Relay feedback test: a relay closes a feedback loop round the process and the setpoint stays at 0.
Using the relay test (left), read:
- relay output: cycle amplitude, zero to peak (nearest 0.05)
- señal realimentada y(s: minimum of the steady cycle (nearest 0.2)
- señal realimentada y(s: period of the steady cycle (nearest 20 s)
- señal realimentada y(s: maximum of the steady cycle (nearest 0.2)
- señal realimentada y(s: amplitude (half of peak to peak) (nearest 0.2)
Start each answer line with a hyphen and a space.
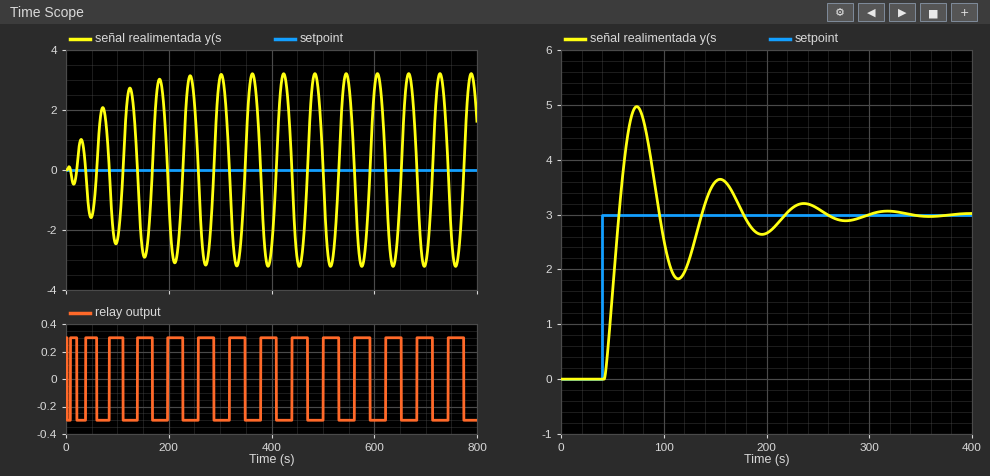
- 0.30
- -3.2
- 60 s
- 3.2
- 3.2
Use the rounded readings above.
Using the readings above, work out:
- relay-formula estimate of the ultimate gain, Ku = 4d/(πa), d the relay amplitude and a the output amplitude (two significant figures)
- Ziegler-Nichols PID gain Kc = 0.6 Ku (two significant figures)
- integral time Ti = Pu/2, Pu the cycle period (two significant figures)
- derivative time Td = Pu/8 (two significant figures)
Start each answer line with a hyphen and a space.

- 0.12
- 0.072
- 30 s
- 7.5 s
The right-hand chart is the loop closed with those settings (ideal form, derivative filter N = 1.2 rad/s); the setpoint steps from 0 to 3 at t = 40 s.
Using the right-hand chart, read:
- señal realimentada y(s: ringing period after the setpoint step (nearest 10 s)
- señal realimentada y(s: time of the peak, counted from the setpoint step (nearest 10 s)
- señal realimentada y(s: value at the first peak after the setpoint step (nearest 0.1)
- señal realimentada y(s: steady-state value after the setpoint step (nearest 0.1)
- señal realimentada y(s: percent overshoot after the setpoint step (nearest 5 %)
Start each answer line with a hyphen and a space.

- 80 s
- 30 s
- 5.0
- 3.0
- 65 %
